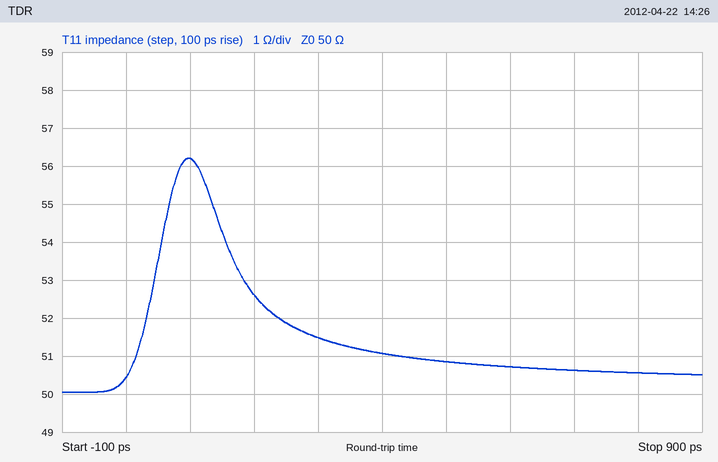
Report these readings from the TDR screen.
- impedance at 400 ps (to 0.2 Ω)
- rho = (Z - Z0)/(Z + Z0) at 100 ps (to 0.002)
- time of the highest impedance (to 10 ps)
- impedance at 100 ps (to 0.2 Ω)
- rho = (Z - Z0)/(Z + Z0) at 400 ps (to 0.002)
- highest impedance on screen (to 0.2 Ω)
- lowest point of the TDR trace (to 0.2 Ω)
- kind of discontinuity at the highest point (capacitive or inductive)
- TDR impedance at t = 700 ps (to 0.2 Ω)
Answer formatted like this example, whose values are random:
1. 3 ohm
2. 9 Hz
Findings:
1. 51.0 Ω
2. +0.058
3. 100 ps
4. 56.2 Ω
5. +0.010
6. 56.2 Ω
7. 50.0 Ω
8. inductive
9. 50.6 Ω
